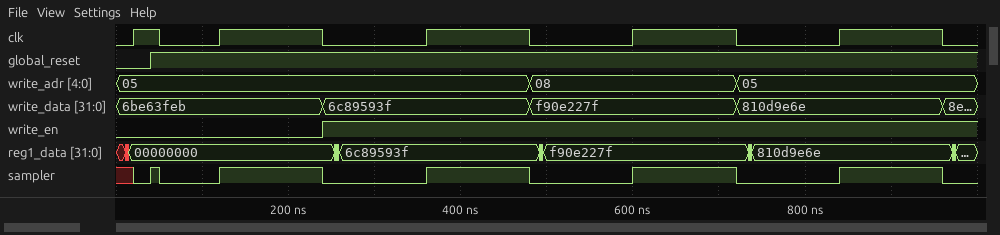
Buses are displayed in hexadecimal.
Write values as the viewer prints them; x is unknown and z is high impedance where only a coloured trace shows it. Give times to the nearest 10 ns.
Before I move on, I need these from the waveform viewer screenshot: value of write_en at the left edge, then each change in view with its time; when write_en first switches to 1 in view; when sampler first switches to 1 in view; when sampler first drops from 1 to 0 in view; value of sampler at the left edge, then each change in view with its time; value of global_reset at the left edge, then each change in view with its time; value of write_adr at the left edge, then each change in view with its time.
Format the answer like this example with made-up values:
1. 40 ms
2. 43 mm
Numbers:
1. 0, 1 at 240 ns
2. 240 ns
3. 40 ns
4. 50 ns
5. x, 0 at 20 ns, 1 at 40 ns, 0 at 50 ns, 1 at 120 ns, 0 at 240 ns, 1 at 360 ns, 0 at 480 ns, 1 at 600 ns, 0 at 720 ns, 1 at 840 ns, 0 at 960 ns
6. 0, 1 at 40 ns
7. 05, 08 at 480 ns, 05 at 720 ns
